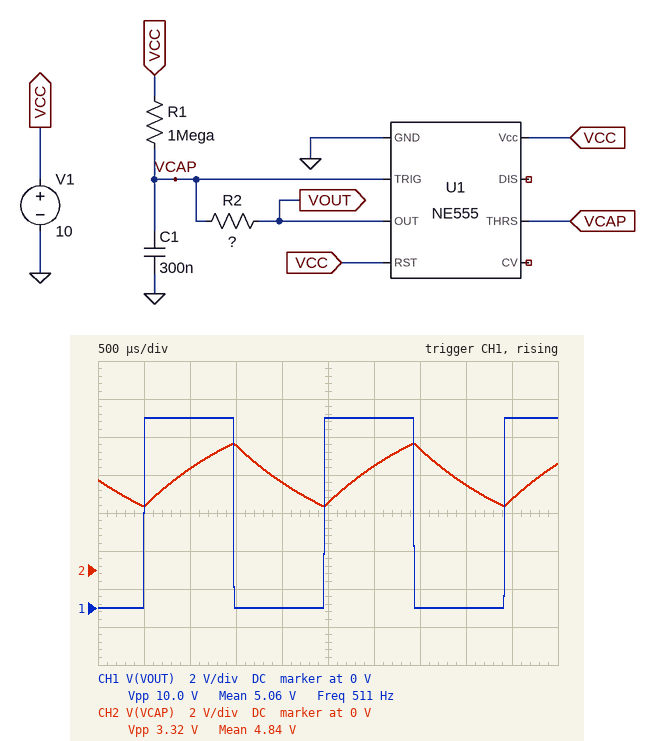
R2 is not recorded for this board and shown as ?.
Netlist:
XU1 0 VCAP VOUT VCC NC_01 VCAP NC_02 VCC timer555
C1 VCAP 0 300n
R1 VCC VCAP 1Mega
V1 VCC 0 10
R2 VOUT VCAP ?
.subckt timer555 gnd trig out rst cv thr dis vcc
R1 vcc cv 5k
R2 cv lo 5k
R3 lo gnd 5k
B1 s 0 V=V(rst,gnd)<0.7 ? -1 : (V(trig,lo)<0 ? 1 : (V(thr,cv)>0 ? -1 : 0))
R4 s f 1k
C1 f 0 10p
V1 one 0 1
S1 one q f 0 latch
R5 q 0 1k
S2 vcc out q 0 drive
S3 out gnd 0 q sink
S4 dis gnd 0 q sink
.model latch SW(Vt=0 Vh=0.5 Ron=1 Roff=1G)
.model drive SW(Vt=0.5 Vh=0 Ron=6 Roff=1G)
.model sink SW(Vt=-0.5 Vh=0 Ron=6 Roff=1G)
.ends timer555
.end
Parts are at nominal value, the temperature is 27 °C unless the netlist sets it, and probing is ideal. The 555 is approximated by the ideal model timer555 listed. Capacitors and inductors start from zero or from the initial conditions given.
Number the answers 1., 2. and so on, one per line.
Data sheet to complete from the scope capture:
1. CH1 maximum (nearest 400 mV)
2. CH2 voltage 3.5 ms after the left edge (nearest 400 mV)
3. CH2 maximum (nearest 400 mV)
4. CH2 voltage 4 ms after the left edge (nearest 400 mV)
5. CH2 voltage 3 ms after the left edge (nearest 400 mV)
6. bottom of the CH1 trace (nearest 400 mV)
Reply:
1. 10.0 V
2. 6.4 V
3. 6.8 V
4. 4.4 V
5. 5.6 V
6. 0 V
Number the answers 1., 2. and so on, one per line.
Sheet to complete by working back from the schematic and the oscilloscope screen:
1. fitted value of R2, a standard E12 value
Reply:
1. 4.7 kΩ
